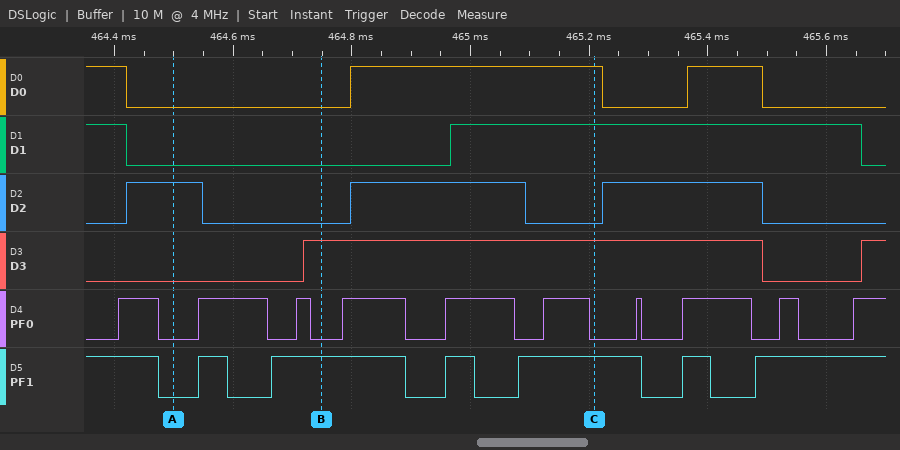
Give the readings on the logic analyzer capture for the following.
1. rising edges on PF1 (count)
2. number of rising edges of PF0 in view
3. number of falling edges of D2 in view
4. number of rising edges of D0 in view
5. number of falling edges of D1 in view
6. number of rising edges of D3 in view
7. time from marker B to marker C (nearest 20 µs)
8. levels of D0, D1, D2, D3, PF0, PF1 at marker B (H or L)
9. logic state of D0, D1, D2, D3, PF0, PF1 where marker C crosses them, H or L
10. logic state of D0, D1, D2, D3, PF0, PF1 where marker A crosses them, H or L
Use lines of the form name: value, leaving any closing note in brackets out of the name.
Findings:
rising edges on PF1: 6
number of rising edges of PF0 in view: 10
number of falling edges of D2 in view: 3
number of rising edges of D0 in view: 2
number of falling edges of D1 in view: 2
number of rising edges of D3 in view: 2
time from marker B to marker C: 460 µs
levels of D0, D1, D2, D3, PF0, PF1 at marker B: D0=L, D1=L, D2=L, D3=H, PF0=L, PF1=H
logic state of D0, D1, D2, D3, PF0, PF1 where marker C crosses them, H or L: D0=H, D1=H, D2=L, D3=H, PF0=L, PF1=H
logic state of D0, D1, D2, D3, PF0, PF1 where marker A crosses them, H or L: D0=L, D1=L, D2=H, D3=L, PF0=L, PF1=L
